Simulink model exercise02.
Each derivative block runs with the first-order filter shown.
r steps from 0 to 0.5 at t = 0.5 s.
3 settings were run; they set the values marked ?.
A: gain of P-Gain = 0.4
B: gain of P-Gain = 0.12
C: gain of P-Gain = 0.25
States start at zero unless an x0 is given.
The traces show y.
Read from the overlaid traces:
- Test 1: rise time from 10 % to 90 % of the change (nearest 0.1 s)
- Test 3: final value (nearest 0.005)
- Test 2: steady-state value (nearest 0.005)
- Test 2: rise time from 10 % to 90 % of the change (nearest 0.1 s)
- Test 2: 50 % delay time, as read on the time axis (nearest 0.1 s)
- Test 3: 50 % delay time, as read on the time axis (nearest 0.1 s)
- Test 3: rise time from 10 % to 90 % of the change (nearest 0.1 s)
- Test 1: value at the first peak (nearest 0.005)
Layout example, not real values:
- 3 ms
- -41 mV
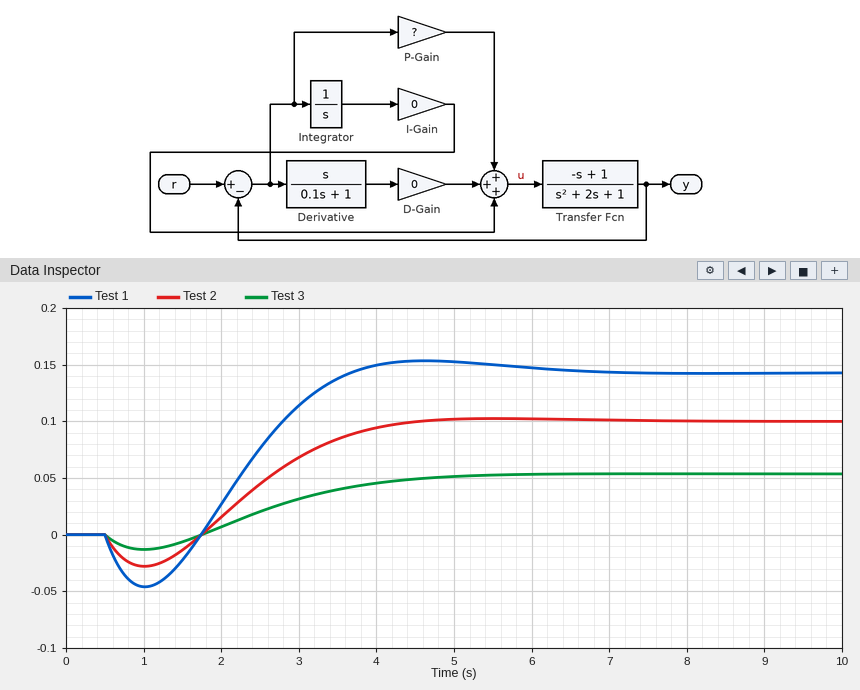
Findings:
- 1.4 s
- 0.055
- 0.100
- 1.8 s
- 2.6 s
- 2.8 s
- 2.4 s
- 0.155
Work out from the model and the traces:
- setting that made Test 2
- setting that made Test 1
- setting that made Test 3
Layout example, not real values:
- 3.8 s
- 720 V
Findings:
- C
- A
- B
